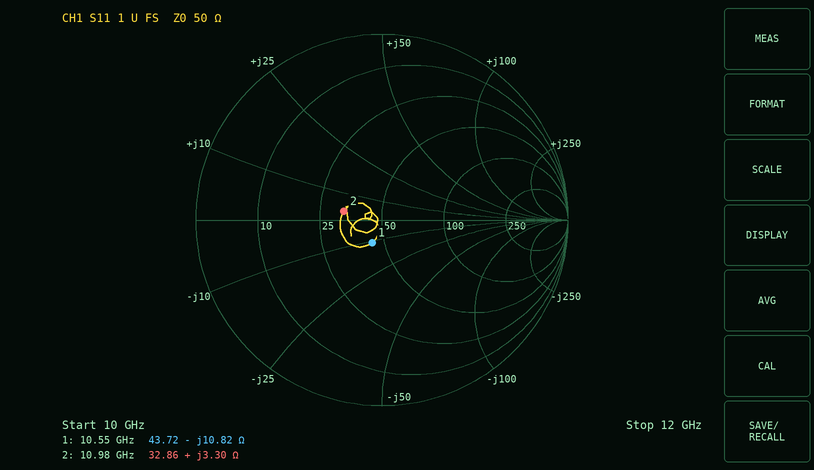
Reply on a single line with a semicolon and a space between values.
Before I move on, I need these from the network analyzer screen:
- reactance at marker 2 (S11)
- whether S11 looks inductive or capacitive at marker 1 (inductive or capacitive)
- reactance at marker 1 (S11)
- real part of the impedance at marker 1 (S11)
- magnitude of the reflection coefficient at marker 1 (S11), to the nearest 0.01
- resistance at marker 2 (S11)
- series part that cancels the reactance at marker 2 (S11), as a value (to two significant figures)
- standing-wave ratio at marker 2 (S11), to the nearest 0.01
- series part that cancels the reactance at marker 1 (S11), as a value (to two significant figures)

+3.30 Ω; capacitive; -10.82 Ω; 43.72 Ω; 0.13; 32.86 Ω; 4.4 pF; 1.53; 160 pH
